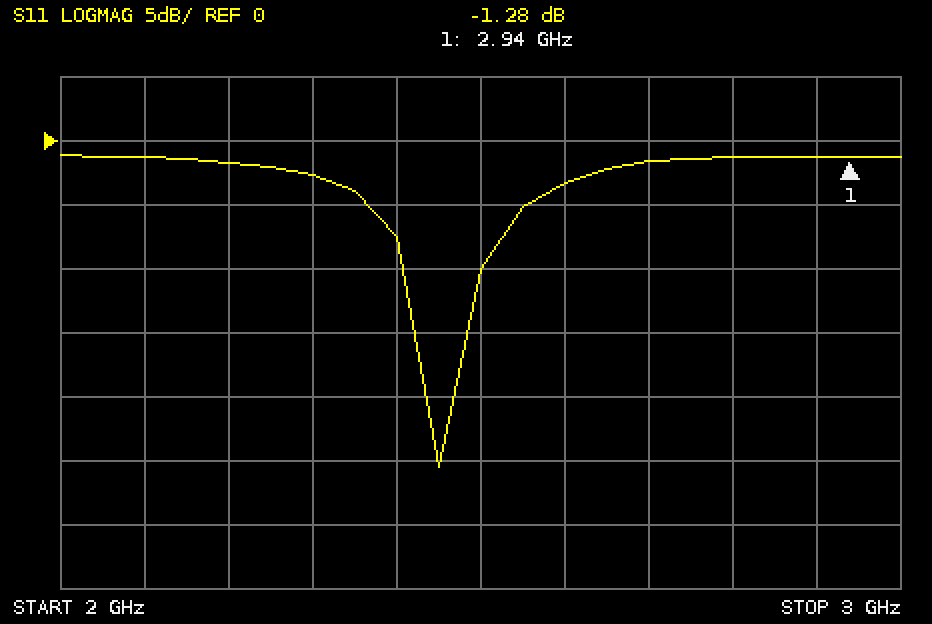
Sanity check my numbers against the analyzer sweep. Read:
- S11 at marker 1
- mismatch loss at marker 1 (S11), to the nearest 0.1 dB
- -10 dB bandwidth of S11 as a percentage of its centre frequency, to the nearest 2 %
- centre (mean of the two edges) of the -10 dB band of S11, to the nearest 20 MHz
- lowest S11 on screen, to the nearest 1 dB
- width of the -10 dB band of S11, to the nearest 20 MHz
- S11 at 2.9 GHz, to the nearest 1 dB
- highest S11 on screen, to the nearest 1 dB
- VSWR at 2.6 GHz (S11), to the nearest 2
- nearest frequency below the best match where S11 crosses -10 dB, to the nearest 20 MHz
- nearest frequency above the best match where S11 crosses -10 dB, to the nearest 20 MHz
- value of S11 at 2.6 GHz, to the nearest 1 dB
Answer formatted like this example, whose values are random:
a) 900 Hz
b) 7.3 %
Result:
a) -1.28 dB
b) 5.9 dB
c) 4 %
d) 2.46 GHz
e) -25 dB
f) 100 MHz
g) -1 dB
h) -1 dB
i) 6
j) 2.40 GHz
k) 2.50 GHz
l) -3 dB
